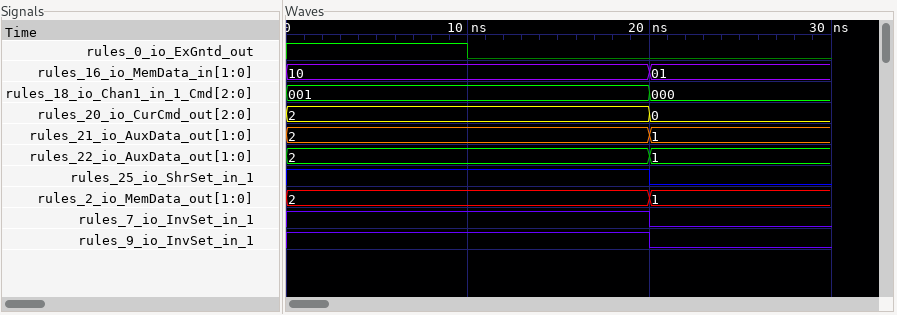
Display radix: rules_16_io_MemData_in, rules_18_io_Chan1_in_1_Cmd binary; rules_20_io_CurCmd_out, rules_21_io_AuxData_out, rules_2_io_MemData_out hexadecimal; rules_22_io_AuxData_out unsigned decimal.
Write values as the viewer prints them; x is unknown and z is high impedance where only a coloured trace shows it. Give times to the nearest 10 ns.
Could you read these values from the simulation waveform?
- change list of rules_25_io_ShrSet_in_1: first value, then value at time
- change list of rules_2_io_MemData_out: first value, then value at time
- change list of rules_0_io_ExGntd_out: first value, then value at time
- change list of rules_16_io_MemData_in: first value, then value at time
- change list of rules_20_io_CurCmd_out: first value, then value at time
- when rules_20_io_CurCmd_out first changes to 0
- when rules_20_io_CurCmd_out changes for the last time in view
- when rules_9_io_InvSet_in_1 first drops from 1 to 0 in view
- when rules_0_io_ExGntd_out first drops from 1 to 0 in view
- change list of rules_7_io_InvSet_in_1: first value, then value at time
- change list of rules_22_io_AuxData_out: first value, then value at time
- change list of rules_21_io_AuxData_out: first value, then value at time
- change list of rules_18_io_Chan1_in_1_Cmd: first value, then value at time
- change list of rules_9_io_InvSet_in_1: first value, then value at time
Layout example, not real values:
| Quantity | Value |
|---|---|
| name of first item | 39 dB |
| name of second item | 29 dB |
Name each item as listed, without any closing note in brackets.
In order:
| Quantity | Value |
|---|---|
| change list of rules_25_io_ShrSet_in_1: first value, then value at time | 1, 0 at 20 ns |
| change list of rules_2_io_MemData_out: first value, then value at time | 2, 1 at 20 ns |
| change list of rules_0_io_ExGntd_out: first value, then value at time | 1, 0 at 10 ns |
| change list of rules_16_io_MemData_in: first value, then value at time | 10, 01 at 20 ns |
| change list of rules_20_io_CurCmd_out: first value, then value at time | 2, 0 at 20 ns |
| when rules_20_io_CurCmd_out first changes to 0 | 20 ns |
| when rules_20_io_CurCmd_out changes for the last time in view | 20 ns |
| when rules_9_io_InvSet_in_1 first drops from 1 to 0 in view | 20 ns |
| when rules_0_io_ExGntd_out first drops from 1 to 0 in view | 10 ns |
| change list of rules_7_io_InvSet_in_1: first value, then value at time | 1, 0 at 20 ns |
| change list of rules_22_io_AuxData_out: first value, then value at time | 2, 1 at 20 ns |
| change list of rules_21_io_AuxData_out: first value, then value at time | 2, 1 at 20 ns |
| change list of rules_18_io_Chan1_in_1_Cmd: first value, then value at time | 001, 000 at 20 ns |
| change list of rules_9_io_InvSet_in_1: first value, then value at time | 1, 0 at 20 ns |
